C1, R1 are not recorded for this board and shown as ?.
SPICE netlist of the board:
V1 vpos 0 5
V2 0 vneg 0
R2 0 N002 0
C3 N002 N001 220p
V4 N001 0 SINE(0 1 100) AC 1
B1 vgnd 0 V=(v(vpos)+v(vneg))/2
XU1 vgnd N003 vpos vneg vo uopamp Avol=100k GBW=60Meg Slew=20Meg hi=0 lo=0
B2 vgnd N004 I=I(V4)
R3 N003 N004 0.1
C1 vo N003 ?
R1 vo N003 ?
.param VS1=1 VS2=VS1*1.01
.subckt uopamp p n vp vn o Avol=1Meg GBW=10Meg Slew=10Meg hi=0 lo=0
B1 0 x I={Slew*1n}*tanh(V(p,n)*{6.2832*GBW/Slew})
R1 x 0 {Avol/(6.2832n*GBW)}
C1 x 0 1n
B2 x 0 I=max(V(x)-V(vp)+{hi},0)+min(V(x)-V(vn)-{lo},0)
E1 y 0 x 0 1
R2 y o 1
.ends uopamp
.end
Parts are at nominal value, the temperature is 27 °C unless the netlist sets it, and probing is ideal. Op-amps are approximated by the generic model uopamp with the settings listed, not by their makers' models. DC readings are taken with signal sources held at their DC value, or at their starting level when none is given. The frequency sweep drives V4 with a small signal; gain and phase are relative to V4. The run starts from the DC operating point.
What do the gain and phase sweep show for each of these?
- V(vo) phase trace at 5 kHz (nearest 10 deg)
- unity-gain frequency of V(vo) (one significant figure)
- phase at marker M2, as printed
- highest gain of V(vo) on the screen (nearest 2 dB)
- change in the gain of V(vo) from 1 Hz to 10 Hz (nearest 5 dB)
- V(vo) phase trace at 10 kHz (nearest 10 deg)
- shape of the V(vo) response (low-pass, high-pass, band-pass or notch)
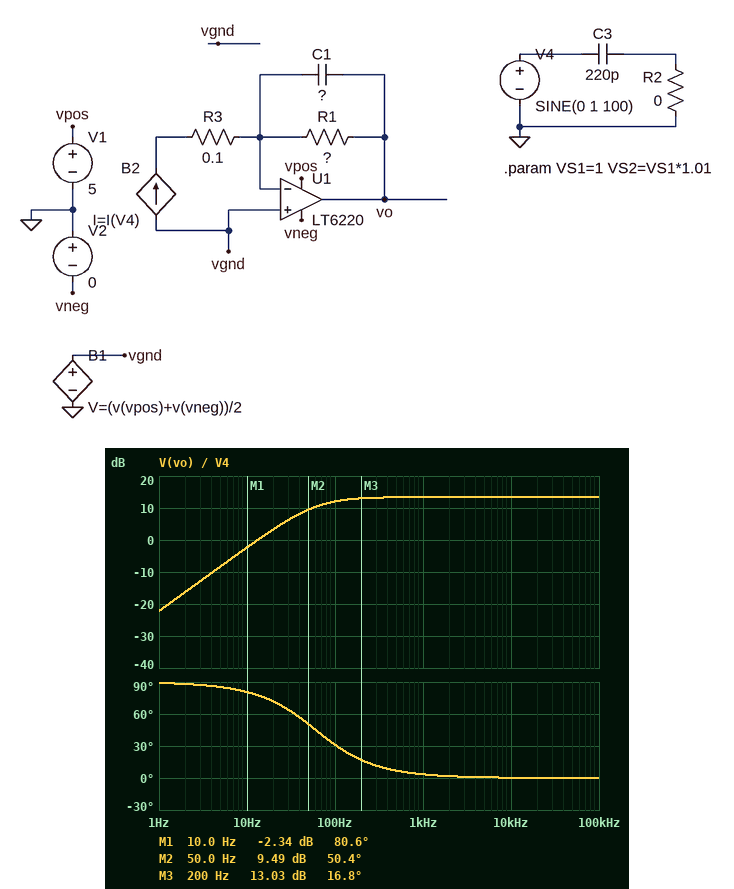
0 deg
10 Hz
50.4 deg
14 dB
20 dB
0 deg
high-pass
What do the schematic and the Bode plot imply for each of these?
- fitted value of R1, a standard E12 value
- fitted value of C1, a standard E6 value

56 MΩ
47 pF
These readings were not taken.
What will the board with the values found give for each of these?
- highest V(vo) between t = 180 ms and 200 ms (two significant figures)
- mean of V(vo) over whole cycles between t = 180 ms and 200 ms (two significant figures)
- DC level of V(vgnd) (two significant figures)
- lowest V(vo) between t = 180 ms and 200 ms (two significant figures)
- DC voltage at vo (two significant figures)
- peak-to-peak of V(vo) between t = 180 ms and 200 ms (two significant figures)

5.0 V
2.5 V
2.5 V
-20 mV
2.5 V
5.0 V
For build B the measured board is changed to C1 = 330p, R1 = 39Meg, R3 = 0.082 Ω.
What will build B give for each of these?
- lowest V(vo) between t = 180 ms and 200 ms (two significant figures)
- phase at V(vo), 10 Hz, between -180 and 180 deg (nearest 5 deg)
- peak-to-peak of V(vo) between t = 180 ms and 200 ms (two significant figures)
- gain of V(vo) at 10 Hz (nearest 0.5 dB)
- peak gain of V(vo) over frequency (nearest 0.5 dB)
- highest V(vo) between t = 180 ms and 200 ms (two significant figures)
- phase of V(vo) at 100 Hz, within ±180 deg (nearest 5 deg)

1.8 V
50 deg
1.3 V
-7.5 dB
-3.5 dB
3.2 V
5 deg
